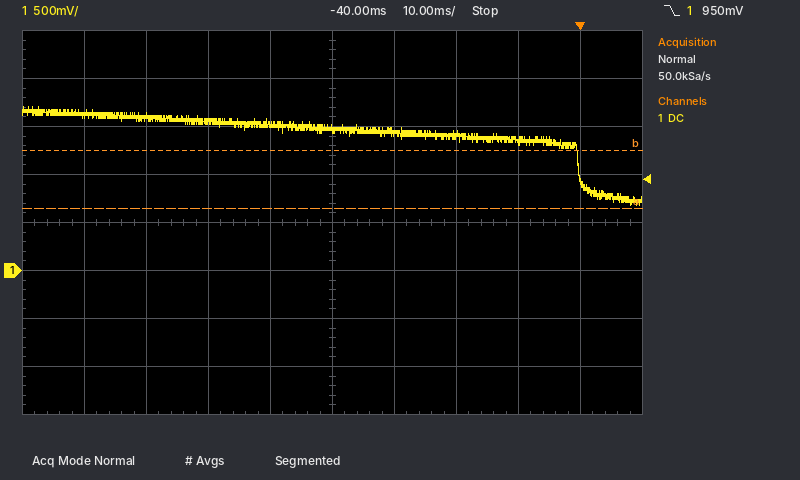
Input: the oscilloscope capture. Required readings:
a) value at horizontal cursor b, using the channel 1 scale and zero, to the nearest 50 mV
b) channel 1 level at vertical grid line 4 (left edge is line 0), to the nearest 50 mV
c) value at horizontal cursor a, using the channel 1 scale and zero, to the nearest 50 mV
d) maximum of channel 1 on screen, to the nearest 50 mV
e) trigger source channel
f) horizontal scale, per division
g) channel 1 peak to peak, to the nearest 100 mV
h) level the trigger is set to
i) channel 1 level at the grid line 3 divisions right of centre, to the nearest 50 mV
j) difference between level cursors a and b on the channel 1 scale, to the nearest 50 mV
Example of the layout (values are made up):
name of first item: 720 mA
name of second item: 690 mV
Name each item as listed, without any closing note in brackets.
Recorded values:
value at horizontal cursor b, using the channel 1 scale and zero, to the nearest 50 mV: 1.25 V
channel 1 level at vertical grid line 4 (left edge is line 0), to the nearest 50 mV: 1.50 V
value at horizontal cursor a, using the channel 1 scale and zero, to the nearest 50 mV: 650 mV
maximum of channel 1 on screen, to the nearest 50 mV: 1.70 V
trigger source channel: channel 1
horizontal scale, per division: 10 ms
channel 1 peak to peak, to the nearest 100 mV: 1.00 V
level the trigger is set to: 950 mV
channel 1 level at the grid line 3 divisions right of centre, to the nearest 50 mV: 1.35 V
difference between level cursors a and b on the channel 1 scale, to the nearest 50 mV: 600 mV
